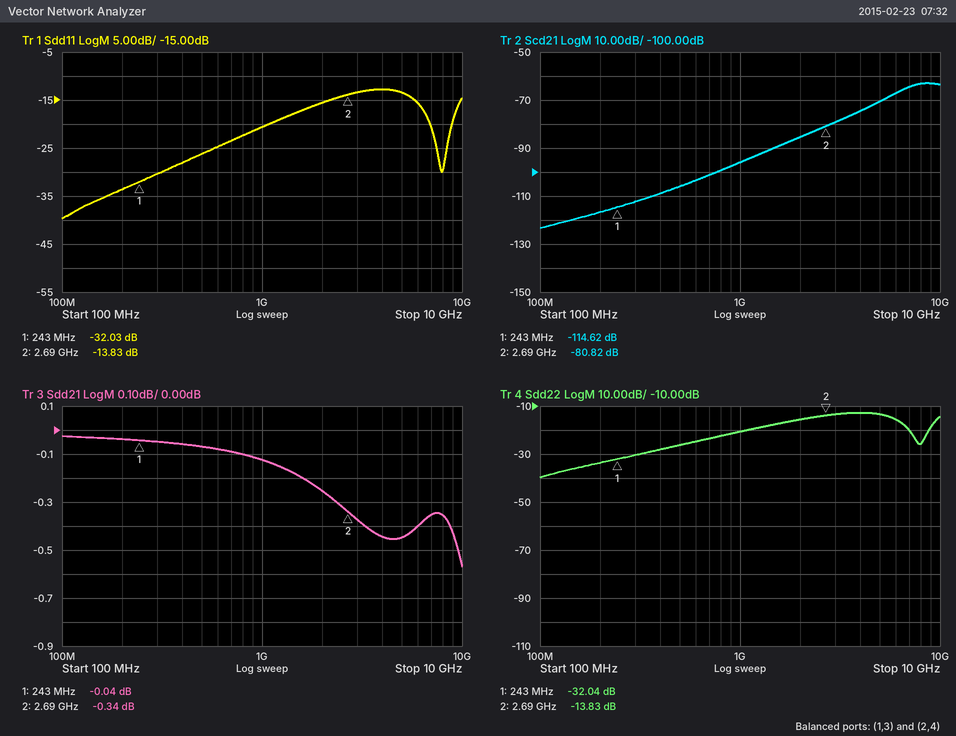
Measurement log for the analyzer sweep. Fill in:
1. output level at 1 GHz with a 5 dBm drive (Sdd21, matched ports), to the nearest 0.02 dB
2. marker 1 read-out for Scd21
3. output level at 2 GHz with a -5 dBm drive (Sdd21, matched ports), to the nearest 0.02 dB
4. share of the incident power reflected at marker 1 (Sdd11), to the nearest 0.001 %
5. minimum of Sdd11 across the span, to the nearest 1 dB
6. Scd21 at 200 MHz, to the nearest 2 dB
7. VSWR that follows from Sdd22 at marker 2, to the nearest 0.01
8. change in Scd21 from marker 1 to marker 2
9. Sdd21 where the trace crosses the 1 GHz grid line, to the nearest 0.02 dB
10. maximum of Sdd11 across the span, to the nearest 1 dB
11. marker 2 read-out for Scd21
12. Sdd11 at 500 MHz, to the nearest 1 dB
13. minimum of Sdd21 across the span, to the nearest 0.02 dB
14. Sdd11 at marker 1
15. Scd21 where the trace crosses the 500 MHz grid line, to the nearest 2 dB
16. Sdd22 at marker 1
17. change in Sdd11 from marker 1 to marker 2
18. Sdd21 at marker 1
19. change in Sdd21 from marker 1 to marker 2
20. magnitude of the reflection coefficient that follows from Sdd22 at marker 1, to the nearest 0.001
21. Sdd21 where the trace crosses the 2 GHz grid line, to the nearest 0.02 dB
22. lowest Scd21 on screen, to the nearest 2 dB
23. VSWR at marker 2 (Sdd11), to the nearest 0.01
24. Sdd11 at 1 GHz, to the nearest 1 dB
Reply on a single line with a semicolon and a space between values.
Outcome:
4.88 dBm; -114.62 dB; -5.26 dBm; 0.063 %; -40 dB; -116 dB; 1.51; 33.80 dB; -0.12 dB; -13 dB; -80.82 dB; -26 dB; -0.56 dB; -32.03 dB; -106 dB; -32.04 dB; 18.20 dB; -0.04 dB; -0.30 dB; 0.025; -0.26 dB; -124 dB; 1.51; -21 dB
